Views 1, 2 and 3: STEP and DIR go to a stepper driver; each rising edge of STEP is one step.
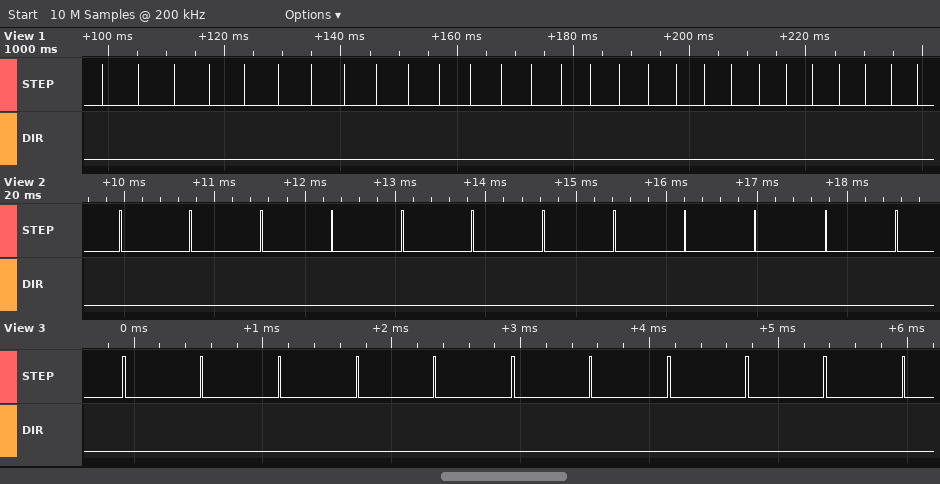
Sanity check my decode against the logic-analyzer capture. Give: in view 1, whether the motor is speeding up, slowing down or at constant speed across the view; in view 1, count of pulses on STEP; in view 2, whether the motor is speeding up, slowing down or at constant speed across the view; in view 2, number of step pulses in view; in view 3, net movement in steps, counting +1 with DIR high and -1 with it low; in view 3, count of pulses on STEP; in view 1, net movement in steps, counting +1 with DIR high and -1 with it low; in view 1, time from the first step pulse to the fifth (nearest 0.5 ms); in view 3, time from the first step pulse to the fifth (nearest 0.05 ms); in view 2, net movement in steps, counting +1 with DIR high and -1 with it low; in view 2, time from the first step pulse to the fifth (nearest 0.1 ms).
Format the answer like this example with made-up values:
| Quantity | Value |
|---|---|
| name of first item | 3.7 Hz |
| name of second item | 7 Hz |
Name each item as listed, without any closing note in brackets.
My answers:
| Quantity | Value |
|---|---|
| in view 1, whether the motor is speeding up, slowing down or at constant speed across the view | speeding up |
| in view 1, count of pulses on STEP | 28 |
| in view 2, whether the motor is speeding up, slowing down or at constant speed across the view | constant speed |
| in view 2, number of step pulses in view | 12 |
| in view 3, net movement in steps, counting +1 with DIR high and -1 with it low | -11 |
| in view 3, count of pulses on STEP | 11 |
| in view 1, net movement in steps, counting +1 with DIR high and -1 with it low | -28 |
| in view 1, time from the first step pulse to the fifth | 24.5 ms |
| in view 3, time from the first step pulse to the fifth | 2.40 ms |
| in view 2, net movement in steps, counting +1 with DIR high and -1 with it low | -12 |
| in view 2, time from the first step pulse to the fifth | 3.1 ms |
